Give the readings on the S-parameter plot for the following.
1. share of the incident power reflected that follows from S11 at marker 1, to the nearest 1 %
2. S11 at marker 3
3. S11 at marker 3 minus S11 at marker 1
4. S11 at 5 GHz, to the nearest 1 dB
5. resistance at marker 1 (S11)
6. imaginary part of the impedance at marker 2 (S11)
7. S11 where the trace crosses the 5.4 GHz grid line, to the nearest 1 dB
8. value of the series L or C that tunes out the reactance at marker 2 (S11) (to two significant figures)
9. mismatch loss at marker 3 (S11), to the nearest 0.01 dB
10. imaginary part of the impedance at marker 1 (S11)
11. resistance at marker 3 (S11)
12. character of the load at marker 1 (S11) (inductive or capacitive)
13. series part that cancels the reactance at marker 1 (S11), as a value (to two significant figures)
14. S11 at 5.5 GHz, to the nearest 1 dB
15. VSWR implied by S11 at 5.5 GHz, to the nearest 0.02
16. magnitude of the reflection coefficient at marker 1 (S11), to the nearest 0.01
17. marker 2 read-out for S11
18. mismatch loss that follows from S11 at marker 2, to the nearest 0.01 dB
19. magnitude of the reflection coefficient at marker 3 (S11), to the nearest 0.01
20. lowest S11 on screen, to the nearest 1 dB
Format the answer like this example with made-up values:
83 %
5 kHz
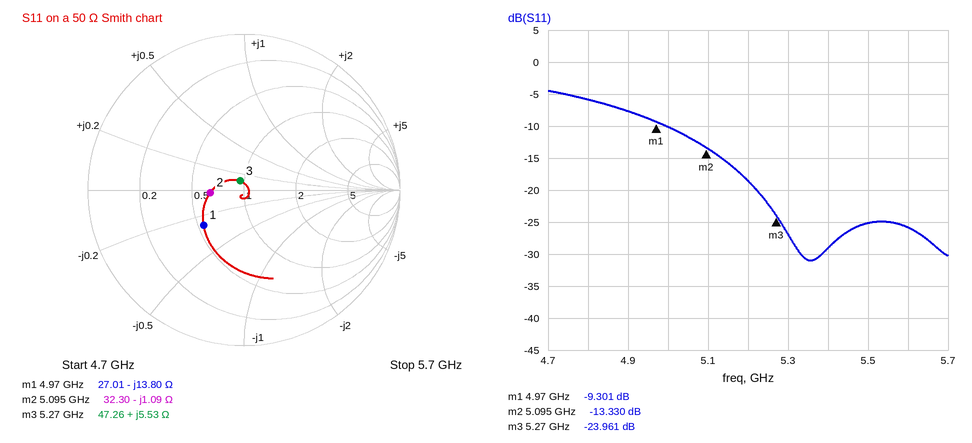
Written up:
12 %
-23.961 dB
-14.660 dB
-10 dB
27.01 Ω
-1.09 Ω
-29 dB
34 pH
0.02 dB
-13.80 Ω
47.26 Ω
capacitive
440 pH
-25 dB
1.12
0.34
-13.330 dB
0.21 dB
0.06
-31 dB
